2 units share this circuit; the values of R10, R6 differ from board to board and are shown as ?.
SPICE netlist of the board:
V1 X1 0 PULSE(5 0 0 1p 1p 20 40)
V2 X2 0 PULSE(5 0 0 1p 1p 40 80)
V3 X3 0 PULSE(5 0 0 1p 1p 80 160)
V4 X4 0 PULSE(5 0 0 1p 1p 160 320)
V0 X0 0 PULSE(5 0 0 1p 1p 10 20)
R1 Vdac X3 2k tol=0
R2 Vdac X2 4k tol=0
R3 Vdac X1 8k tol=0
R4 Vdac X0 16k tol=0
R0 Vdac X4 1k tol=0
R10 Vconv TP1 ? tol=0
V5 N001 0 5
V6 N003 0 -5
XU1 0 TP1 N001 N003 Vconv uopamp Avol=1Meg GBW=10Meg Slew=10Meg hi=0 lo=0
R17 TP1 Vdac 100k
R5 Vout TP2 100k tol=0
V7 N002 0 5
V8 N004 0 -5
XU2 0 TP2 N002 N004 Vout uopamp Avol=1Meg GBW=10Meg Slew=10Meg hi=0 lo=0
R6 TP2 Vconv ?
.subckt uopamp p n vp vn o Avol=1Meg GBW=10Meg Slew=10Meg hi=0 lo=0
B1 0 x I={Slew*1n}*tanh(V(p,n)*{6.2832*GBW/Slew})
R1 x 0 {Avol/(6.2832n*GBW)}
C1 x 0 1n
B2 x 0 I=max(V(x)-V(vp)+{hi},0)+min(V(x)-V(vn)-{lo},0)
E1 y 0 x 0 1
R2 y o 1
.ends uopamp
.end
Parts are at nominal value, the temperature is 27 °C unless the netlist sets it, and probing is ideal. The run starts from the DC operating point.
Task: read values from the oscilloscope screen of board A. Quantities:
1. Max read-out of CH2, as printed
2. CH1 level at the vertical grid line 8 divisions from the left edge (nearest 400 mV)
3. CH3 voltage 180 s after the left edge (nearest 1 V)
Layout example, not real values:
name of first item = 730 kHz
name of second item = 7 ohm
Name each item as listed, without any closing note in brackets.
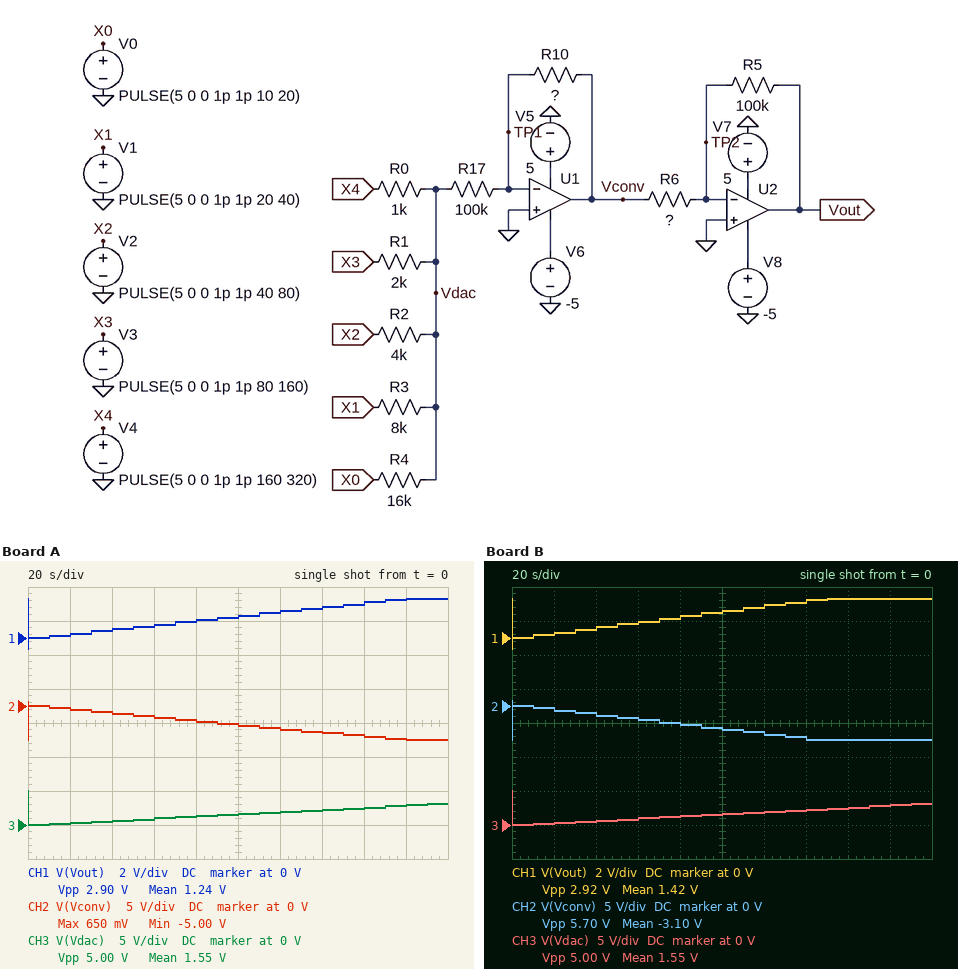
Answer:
Max read-out of CH2, as printed = 650 mV
CH1 level at the vertical grid line 8 divisions from the left edge = 2.0 V
CH3 voltage 180 s after the left edge = 3 V
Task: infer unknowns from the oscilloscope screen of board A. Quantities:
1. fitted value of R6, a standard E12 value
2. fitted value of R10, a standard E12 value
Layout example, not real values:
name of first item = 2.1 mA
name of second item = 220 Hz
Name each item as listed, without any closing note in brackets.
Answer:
fitted value of R6, a standard E12 value = 220 kΩ
fitted value of R10, a standard E12 value = 180 kΩ
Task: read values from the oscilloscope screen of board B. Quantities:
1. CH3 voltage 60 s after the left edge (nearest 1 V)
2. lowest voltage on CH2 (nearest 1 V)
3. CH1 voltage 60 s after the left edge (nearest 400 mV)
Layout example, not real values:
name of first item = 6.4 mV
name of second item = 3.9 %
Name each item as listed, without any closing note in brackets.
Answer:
CH3 voltage 60 s after the left edge = 1 V
lowest voltage on CH2 = -5 V
CH1 voltage 60 s after the left edge = 800 mV
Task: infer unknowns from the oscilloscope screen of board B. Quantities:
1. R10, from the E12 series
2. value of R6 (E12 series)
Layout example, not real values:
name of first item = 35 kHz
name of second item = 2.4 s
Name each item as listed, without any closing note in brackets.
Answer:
R10, from the E12 series = 220 kΩ
value of R6 = 220 kΩ
